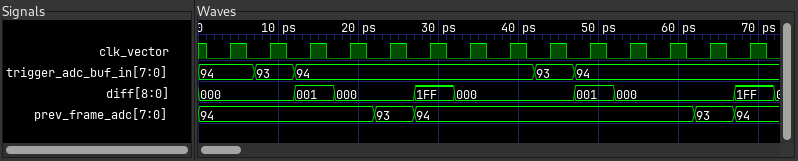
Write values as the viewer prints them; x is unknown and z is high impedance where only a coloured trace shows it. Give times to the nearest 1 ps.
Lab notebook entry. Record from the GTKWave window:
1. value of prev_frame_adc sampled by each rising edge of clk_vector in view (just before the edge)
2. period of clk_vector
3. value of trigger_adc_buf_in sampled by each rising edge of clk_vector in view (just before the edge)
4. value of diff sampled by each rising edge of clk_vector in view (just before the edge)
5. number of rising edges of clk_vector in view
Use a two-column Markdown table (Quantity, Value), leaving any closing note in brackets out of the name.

| Quantity | Value |
|---|---|
| value of prev_frame_adc sampled by each rising edge of clk_vector in view | 94, 94, 94, 94, 93, 94, 94, 94, 94, 94, 94, 94, 93, 94 |
| period of clk_vector | 5 ps |
| value of trigger_adc_buf_in sampled by each rising edge of clk_vector in view | 94, 93, 94, 94, 94, 94, 94, 94, 93, 94, 94, 94, 94, 94 |
| value of diff sampled by each rising edge of clk_vector in view | 000, 000, 001, 000, 000, 1FF, 000, 000, 000, 001, 000, 000, 000, 1FF |
| number of rising edges of clk_vector in view | 14 |
